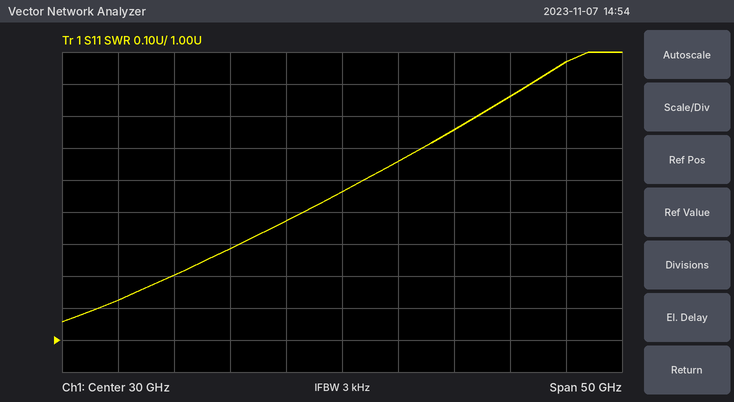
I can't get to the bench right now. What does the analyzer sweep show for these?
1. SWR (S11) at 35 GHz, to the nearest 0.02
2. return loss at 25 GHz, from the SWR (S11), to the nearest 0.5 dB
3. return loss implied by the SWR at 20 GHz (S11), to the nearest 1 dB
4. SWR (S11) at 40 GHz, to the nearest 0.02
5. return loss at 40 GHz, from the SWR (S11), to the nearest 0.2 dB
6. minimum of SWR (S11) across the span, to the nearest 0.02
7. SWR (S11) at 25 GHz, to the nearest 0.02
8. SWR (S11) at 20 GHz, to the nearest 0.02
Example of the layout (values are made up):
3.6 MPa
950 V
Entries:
1.56
16.0 dB
18 dB
1.66
12.2 dB
1.06
1.38
1.28
